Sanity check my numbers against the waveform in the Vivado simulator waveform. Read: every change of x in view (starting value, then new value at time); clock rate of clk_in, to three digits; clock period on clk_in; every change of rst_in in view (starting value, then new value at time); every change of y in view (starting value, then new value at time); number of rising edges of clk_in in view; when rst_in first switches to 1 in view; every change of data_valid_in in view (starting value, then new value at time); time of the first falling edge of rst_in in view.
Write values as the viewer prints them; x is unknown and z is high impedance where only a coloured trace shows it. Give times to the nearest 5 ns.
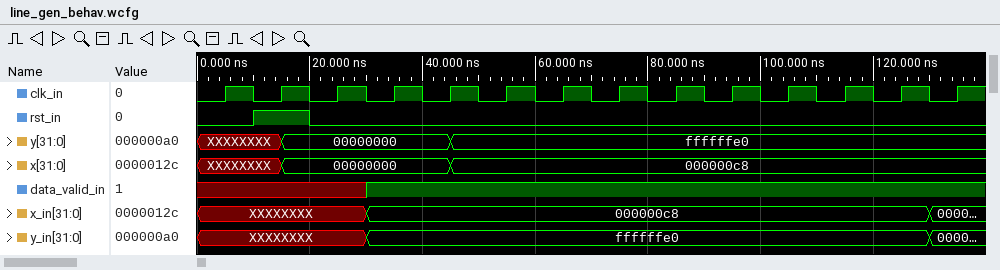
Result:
XXXXXXXX, 00000000 at 15 ns, 000000c8 at 45 ns
100 MHz
10 ns
0, 1 at 10 ns, 0 at 20 ns
XXXXXXXX, 00000000 at 15 ns, ffffffe0 at 45 ns
14
10 ns
x, 1 at 30 ns
20 ns
